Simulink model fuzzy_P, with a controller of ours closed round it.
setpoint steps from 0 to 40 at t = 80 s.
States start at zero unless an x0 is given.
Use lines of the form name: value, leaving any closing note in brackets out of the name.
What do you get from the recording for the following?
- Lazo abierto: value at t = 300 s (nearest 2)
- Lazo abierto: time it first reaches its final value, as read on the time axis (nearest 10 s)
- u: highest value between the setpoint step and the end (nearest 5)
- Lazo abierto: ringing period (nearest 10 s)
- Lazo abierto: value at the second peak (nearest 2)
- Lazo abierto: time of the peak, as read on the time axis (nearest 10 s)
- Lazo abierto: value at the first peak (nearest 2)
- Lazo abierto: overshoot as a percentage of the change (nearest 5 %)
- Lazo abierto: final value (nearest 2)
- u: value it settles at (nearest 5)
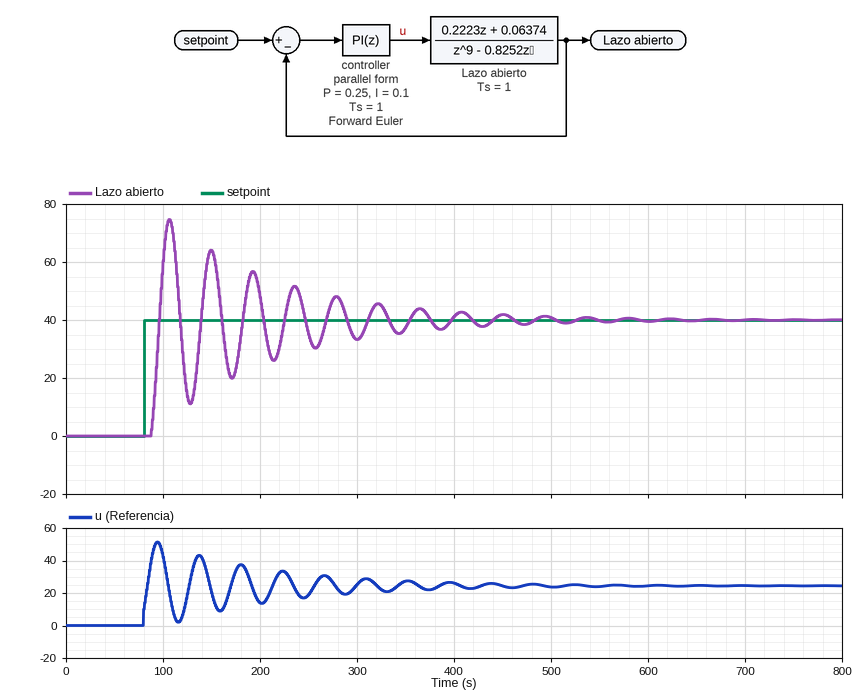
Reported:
Lazo abierto: value at t = 300 s: 34
Lazo abierto: time it first reaches its final value, as read on the time axis: 100 s
u: highest value between the setpoint step and the end: 50
Lazo abierto: ringing period: 40 s
Lazo abierto: value at the second peak: 64
Lazo abierto: time of the peak, as read on the time axis: 110 s
Lazo abierto: value at the first peak: 74
Lazo abierto: overshoot as a percentage of the change: 85 %
Lazo abierto: final value: 40
u: value it settles at: 25
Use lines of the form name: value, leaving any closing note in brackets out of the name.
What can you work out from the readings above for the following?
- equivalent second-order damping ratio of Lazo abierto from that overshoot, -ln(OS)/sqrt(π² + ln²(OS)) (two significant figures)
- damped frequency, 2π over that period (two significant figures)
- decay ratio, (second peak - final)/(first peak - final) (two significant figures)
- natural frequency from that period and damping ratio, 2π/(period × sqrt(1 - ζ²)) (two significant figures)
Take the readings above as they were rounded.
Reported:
equivalent second-order damping ratio of Lazo abierto from that overshoot, -ln(OS)/sqrt(π² + ln²(OS)): 0.052
damped frequency, 2π over that period: 0.16 rad/s
decay ratio, (second peak - final)/(first peak - final): 0.71
natural frequency from that period and damping ratio, 2π/(period × sqrt(1 - ζ²)): 0.16 rad/s
